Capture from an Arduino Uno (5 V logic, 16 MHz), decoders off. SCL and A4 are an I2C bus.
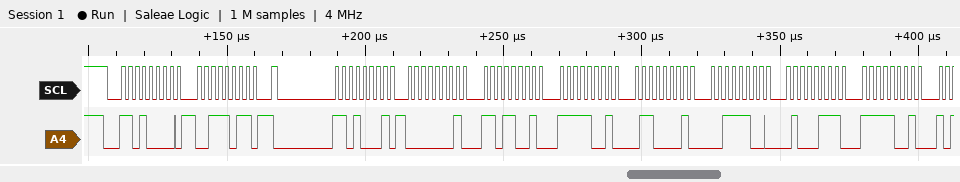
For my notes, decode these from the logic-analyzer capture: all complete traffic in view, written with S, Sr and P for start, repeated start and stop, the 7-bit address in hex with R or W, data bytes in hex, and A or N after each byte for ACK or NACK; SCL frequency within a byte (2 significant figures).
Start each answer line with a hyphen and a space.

- S 68W A 3B A Sr 68R A 01 A D9 A F9 A 61 A 3C A 47 A F9 A
- 400 kHz
